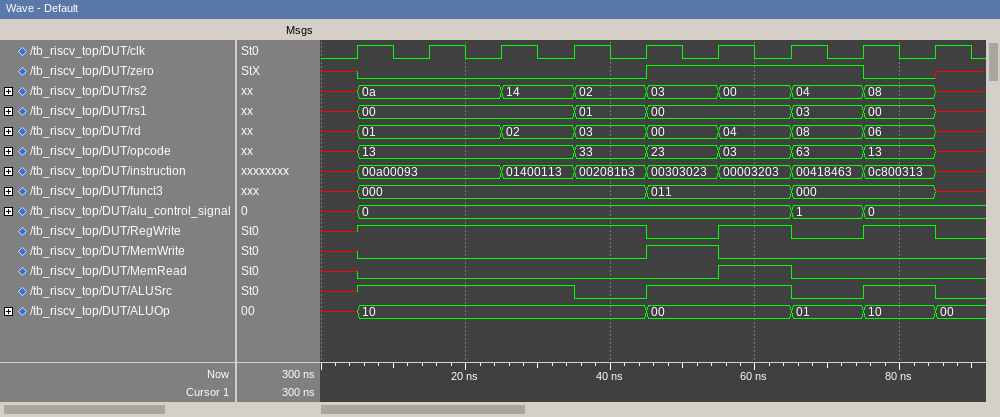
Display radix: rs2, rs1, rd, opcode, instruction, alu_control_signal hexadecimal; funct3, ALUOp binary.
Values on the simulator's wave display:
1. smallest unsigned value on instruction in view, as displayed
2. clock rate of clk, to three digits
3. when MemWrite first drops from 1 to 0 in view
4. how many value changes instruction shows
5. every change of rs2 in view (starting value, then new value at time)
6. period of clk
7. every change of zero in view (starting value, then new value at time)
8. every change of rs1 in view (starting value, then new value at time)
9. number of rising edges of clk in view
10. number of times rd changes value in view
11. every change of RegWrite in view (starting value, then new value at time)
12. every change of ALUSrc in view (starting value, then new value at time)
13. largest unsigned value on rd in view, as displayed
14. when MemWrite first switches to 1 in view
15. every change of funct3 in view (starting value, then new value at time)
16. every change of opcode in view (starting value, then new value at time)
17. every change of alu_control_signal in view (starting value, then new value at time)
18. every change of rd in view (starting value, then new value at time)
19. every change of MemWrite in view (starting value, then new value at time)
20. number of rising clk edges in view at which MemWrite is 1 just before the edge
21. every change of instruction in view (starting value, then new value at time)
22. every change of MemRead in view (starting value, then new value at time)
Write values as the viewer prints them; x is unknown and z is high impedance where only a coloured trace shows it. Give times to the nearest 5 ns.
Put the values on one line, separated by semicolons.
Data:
00003203; 100 MHz; 55 ns; 8; x, 0a at 5 ns, 14 at 25 ns, 02 at 35 ns, 03 at 45 ns, 00 at 55 ns, 04 at 65 ns, 08 at 75 ns, x at 85 ns; 10 ns; x, 0 at 5 ns, 1 at 45 ns, 0 at 75 ns, x at 85 ns; x, 00 at 5 ns, 01 at 35 ns, 00 at 45 ns, 03 at 65 ns, 00 at 75 ns, x at 85 ns; 9; 8; x, 1 at 5 ns, 0 at 45 ns, 1 at 55 ns, 0 at 65 ns, 1 at 75 ns, 0 at 85 ns; x, 1 at 5 ns, 0 at 35 ns, 1 at 45 ns, 0 at 65 ns, 1 at 75 ns, 0 at 85 ns; 08; 45 ns; x, 000 at 5 ns, 011 at 45 ns, 000 at 65 ns, x at 85 ns; x, 13 at 5 ns, 33 at 35 ns, 23 at 45 ns, 03 at 55 ns, 63 at 65 ns, 13 at 75 ns, x at 85 ns; x, 0 at 5 ns, 1 at 65 ns, 0 at 75 ns; x, 01 at 5 ns, 02 at 25 ns, 03 at 35 ns, 00 at 45 ns, 04 at 55 ns, 08 at 65 ns, 06 at 75 ns, x at 85 ns; x, 0 at 5 ns, 1 at 45 ns, 0 at 55 ns; 1; x, 00a00093 at 5 ns, 01400113 at 25 ns, 002081b3 at 35 ns, 00303023 at 45 ns, 00003203 at 55 ns, 00418463 at 65 ns, 0c800313 at 75 ns, x at 85 ns; x, 0 at 5 ns, 1 at 55 ns, 0 at 65 ns
